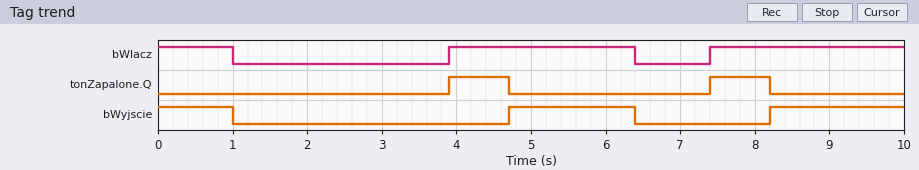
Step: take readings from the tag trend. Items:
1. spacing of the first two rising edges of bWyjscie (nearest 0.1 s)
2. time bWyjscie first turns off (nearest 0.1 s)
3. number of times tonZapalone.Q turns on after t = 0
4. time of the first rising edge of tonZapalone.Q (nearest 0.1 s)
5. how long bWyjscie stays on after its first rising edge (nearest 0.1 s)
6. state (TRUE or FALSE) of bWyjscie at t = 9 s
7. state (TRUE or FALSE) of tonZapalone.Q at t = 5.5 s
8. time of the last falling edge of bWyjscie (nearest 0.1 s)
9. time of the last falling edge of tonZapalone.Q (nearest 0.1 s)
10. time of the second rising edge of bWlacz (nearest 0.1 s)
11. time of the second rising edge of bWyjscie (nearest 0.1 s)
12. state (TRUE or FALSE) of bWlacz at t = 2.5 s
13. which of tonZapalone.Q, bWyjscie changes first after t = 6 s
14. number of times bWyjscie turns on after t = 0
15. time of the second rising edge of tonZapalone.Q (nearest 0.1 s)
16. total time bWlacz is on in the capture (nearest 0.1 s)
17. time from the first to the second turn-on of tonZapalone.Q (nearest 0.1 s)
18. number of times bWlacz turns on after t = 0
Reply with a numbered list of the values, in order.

1. 3.5 s
2. 1.0 s
3. 2
4. 3.9 s
5. 1.7 s
6. TRUE
7. FALSE
8. 6.4 s
9. 8.2 s
10. 7.4 s
11. 8.2 s
12. FALSE
13. bWyjscie
14. 2
15. 7.4 s
16. 6.1 s
17. 3.5 s
18. 2
